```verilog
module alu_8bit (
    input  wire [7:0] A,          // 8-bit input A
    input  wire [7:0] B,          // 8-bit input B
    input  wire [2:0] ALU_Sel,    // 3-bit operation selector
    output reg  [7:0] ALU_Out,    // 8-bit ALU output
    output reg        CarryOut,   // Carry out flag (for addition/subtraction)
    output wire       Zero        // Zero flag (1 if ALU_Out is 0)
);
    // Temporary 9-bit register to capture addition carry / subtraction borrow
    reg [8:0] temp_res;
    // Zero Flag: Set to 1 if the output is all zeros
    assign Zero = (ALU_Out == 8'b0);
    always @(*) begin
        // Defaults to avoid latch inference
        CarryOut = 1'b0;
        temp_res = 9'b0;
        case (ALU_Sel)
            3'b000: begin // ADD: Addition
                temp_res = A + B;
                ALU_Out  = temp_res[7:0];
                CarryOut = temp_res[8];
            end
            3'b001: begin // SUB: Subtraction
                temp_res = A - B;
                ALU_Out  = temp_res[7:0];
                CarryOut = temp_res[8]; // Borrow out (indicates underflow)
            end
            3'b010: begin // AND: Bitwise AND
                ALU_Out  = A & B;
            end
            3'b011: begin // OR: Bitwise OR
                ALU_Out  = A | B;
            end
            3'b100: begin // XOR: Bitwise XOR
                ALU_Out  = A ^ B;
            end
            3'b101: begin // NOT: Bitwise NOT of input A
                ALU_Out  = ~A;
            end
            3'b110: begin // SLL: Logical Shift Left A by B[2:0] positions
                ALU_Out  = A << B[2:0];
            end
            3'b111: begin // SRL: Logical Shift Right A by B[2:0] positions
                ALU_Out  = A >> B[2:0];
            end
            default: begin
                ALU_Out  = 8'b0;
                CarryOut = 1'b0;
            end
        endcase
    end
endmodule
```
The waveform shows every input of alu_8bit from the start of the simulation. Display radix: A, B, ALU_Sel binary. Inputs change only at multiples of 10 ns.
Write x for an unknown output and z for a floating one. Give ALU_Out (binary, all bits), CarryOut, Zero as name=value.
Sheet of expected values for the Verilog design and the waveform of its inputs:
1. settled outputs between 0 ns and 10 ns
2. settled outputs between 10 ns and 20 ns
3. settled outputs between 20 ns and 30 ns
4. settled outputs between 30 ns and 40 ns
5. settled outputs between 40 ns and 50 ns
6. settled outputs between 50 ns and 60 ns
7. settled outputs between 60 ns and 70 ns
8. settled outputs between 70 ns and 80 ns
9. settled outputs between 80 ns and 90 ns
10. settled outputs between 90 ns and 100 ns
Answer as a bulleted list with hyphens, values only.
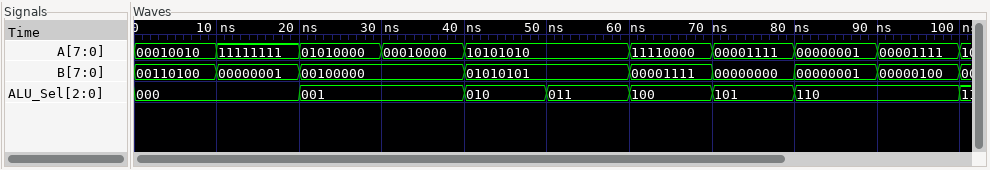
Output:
- ALU_Out=01000110, CarryOut=0, Zero=0
- ALU_Out=00000000, CarryOut=1, Zero=1
- ALU_Out=00110000, CarryOut=0, Zero=0
- ALU_Out=11110000, CarryOut=1, Zero=0
- ALU_Out=00000000, CarryOut=0, Zero=1
- ALU_Out=11111111, CarryOut=0, Zero=0
- ALU_Out=11111111, CarryOut=0, Zero=0
- ALU_Out=11110000, CarryOut=0, Zero=0
- ALU_Out=00000010, CarryOut=0, Zero=0
- ALU_Out=11110000, CarryOut=0, Zero=0
